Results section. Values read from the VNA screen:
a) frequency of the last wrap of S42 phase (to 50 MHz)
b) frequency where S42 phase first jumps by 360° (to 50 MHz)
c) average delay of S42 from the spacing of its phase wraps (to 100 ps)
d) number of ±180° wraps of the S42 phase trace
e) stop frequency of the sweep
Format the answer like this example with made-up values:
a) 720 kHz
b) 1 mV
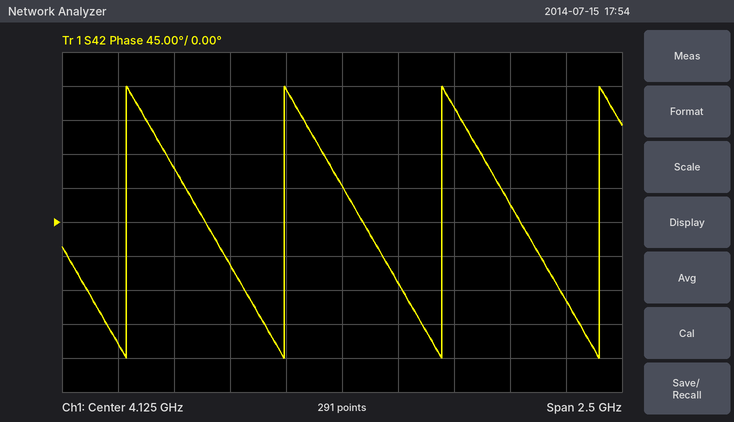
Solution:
a) 5.25 GHz
b) 3.15 GHz
c) 1.4 ns
d) 4
e) 5.375 GHz
